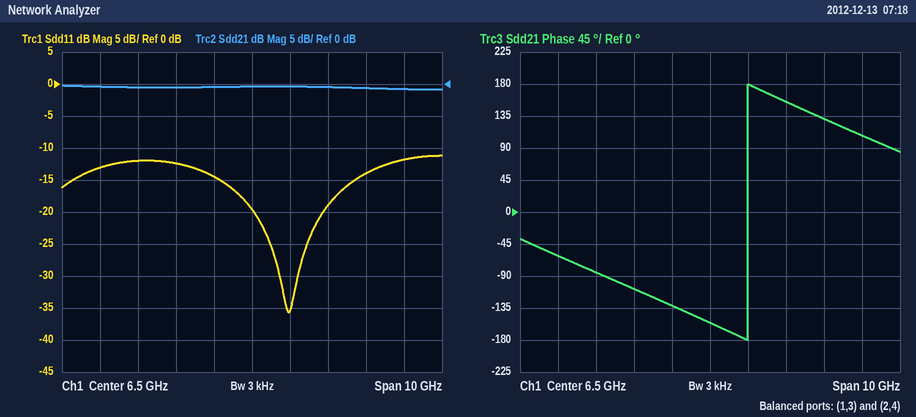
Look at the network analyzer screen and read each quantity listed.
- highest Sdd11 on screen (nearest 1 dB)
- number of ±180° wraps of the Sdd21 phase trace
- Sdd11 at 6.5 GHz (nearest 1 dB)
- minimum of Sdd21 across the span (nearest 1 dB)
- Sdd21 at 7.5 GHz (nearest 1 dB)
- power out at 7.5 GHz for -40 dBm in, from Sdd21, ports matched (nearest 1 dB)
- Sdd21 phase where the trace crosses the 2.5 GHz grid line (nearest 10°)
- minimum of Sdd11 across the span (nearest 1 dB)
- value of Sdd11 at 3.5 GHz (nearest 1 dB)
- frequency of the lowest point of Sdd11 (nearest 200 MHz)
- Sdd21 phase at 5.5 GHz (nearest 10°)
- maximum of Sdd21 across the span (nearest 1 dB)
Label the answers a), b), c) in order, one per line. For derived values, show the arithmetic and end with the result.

a) -11 dB
b) 1
c) -20 dB
d) -1 dB
e) 0 dB
f) -40 dBm + (0 dB) = -40 dBm
g) -60°
h) -36 dB
i) -12 dB
j) 7.4 GHz
k) -130°
l) 0 dB
